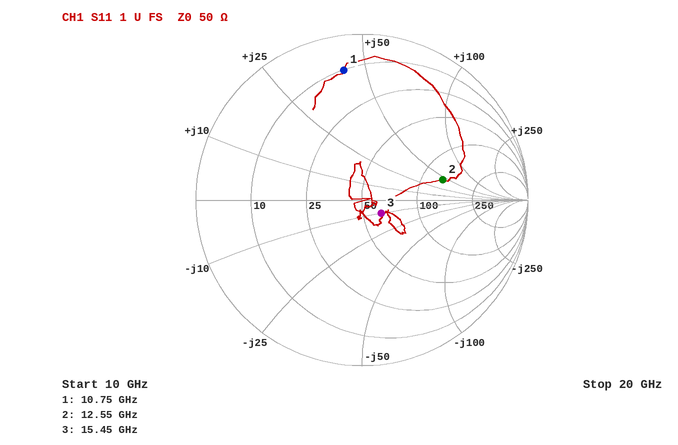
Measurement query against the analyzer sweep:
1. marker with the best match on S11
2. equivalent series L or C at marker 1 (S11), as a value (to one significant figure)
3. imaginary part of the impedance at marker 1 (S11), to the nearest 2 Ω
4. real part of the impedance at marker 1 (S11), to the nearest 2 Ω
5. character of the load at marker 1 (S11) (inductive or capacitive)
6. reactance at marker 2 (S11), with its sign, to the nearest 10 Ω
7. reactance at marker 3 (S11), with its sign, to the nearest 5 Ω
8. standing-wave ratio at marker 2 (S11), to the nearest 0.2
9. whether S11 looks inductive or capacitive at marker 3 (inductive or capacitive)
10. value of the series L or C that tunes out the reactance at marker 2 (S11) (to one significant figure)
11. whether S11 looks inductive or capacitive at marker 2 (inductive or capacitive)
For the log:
marker 3
600 pH
+42 Ω
10 Ω
inductive
+40 Ω
-10 Ω
3.0
capacitive
300 fF
inductive
